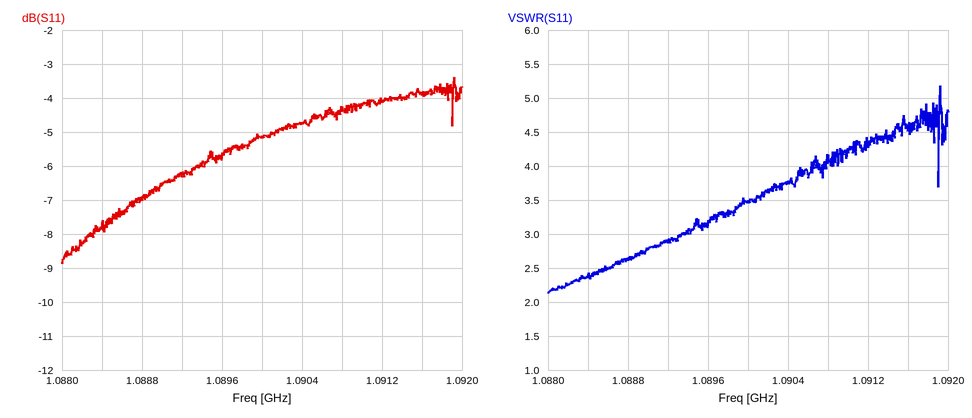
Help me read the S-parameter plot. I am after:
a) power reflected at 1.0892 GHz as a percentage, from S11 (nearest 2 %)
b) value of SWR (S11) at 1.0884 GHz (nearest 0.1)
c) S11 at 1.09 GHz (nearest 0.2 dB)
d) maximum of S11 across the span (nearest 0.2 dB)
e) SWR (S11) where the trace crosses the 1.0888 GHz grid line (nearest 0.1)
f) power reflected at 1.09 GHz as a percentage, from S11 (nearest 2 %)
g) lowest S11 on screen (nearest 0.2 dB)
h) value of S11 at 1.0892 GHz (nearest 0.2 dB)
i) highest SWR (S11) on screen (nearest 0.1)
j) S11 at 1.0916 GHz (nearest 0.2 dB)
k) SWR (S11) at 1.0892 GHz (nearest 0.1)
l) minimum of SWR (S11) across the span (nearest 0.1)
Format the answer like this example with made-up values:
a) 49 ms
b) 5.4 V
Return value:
a) 24 %
b) 2.4
c) -5.2 dB
d) -3.4 dB
e) 2.6
f) 30 %
g) -8.8 dB
h) -6.2 dB
i) 5.2
j) -3.8 dB
k) 2.9
l) 2.1
